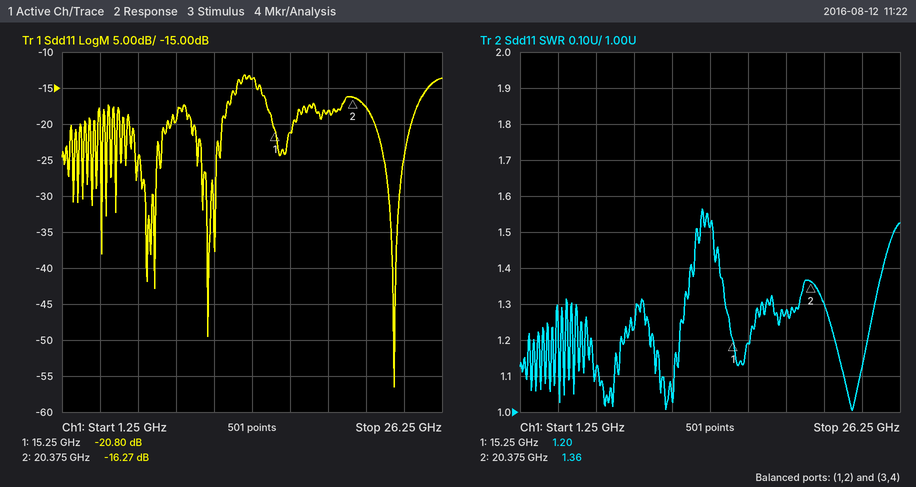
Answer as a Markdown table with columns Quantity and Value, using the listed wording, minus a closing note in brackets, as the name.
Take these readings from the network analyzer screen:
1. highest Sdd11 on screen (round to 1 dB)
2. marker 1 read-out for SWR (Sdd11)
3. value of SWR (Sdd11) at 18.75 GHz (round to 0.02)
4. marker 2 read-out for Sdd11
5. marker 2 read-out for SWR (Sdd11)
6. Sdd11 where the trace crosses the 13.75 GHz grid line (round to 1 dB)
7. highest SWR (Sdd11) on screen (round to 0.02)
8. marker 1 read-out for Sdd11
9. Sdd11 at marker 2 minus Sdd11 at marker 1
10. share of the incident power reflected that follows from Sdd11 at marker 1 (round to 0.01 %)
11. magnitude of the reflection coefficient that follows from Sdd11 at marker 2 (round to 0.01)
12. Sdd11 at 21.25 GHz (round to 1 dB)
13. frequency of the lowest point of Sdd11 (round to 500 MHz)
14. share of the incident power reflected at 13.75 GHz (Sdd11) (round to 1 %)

| Quantity | Value |
|---|---|
| highest Sdd11 on screen | -13 dB |
| marker 1 read-out for SWR | 1.20 |
| value of SWR (Sdd11) at 18.75 GHz | 1.28 |
| marker 2 read-out for Sdd11 | -16.27 dB |
| marker 2 read-out for SWR | 1.36 |
| Sdd11 where the trace crosses the 13.75 GHz grid line | -14 dB |
| highest SWR (Sdd11) on screen | 1.56 |
| marker 1 read-out for Sdd11 | -20.80 dB |
| Sdd11 at marker 2 minus Sdd11 at marker 1 | 4.53 dB |
| share of the incident power reflected that follows from Sdd11 at marker 1 | 0.83 % |
| magnitude of the reflection coefficient that follows from Sdd11 at marker 2 | 0.15 |
| Sdd11 at 21.25 GHz | -18 dB |
| frequency of the lowest point of Sdd11 | 23.0 GHz |
| share of the incident power reflected at 13.75 GHz (Sdd11) | 4 % |
